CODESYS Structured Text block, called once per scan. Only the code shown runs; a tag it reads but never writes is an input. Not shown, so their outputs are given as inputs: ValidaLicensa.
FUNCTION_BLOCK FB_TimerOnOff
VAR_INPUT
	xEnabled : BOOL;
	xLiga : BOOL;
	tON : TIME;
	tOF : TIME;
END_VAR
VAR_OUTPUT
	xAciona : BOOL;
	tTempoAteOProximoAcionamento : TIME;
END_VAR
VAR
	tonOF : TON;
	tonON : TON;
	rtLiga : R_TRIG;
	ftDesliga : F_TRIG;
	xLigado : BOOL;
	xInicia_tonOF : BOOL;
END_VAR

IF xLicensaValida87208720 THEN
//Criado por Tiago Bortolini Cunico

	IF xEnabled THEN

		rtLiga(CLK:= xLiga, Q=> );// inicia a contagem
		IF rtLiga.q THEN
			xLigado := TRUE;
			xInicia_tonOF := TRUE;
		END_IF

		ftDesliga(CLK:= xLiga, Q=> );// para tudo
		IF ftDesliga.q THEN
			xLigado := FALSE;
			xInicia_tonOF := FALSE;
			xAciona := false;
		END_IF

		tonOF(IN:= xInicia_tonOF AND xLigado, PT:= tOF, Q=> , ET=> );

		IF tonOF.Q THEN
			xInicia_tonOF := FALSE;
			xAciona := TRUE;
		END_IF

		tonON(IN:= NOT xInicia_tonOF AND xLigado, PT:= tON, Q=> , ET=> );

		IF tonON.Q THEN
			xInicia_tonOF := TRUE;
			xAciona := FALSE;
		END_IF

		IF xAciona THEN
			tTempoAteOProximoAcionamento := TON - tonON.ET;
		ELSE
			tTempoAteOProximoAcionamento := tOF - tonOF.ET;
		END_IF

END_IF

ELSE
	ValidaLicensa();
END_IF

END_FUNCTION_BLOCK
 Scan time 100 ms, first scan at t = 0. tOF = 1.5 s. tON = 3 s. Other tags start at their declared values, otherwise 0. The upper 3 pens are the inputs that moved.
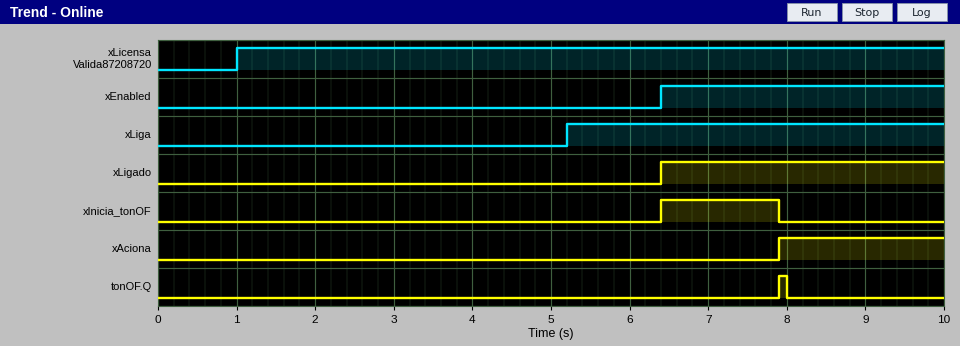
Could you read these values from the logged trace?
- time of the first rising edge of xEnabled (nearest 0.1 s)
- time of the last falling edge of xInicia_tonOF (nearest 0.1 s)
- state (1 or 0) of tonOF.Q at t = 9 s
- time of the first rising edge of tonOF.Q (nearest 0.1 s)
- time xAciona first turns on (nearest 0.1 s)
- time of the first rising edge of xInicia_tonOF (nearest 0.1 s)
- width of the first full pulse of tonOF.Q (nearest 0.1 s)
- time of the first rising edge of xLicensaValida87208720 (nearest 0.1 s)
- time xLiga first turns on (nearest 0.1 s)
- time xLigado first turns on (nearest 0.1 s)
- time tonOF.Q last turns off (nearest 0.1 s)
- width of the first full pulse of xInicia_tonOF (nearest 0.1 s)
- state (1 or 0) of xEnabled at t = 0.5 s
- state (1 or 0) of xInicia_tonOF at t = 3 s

6.4 s
7.9 s
0
7.9 s
7.9 s
6.4 s
0.1 s
1.0 s
5.2 s
6.4 s
8.0 s
1.5 s
0
0
